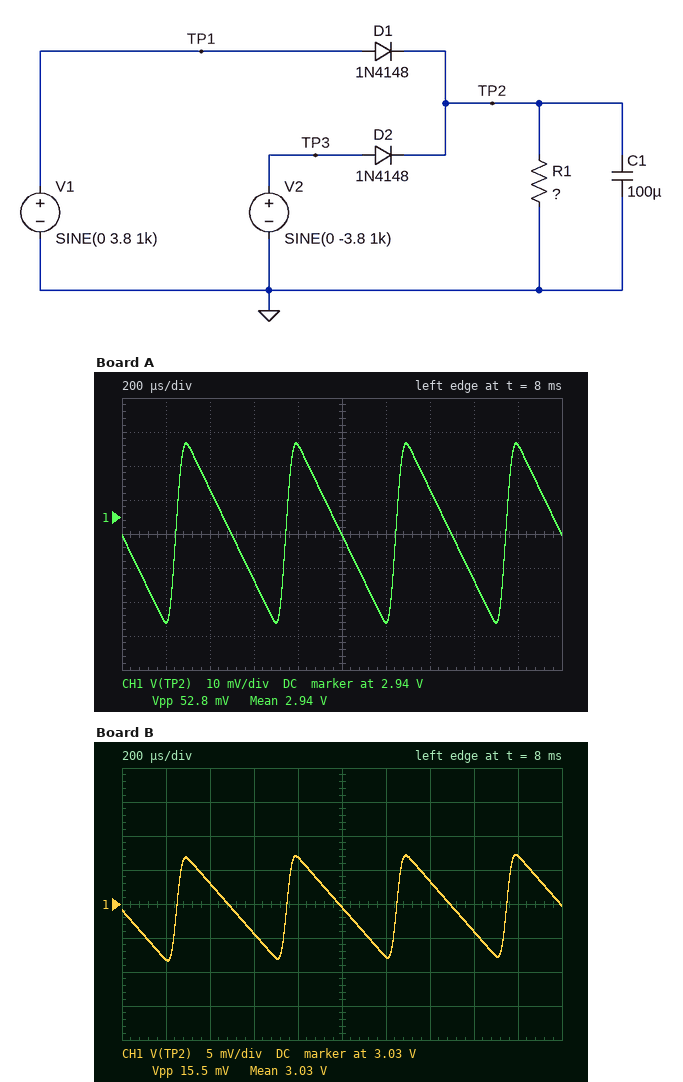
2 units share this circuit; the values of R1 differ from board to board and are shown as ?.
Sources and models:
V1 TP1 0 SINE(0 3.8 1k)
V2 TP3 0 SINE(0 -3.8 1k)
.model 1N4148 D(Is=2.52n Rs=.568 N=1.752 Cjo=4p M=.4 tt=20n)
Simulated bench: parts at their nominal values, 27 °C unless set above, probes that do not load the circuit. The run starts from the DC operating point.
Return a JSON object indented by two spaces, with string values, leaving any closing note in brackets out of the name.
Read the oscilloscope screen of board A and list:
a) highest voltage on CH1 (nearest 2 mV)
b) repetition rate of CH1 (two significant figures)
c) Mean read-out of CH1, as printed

{
  "highest voltage on CH1": "2.962 V",
  "repetition rate of CH1": "2.0 kHz",
  "Mean read-out of CH1, as printed": "2.94 V"
}
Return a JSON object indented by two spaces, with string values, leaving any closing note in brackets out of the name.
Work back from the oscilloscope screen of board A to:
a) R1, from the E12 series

{
  "R1, from the E12 series": "220 Ω"
}
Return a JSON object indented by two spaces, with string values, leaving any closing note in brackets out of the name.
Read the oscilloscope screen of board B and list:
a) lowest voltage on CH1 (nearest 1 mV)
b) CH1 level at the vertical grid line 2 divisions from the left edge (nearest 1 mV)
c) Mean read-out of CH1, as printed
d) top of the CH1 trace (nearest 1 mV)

{
  "lowest voltage on CH1": "3.022 V",
  "CH1 level at the vertical grid line 2 divisions from the left edge": "3.033 V",
  "Mean read-out of CH1, as printed": "3.03 V",
  "top of the CH1 trace": "3.037 V"
}
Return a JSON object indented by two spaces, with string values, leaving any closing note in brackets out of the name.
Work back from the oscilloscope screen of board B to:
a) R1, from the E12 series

{
  "R1, from the E12 series": "820 Ω"
}
